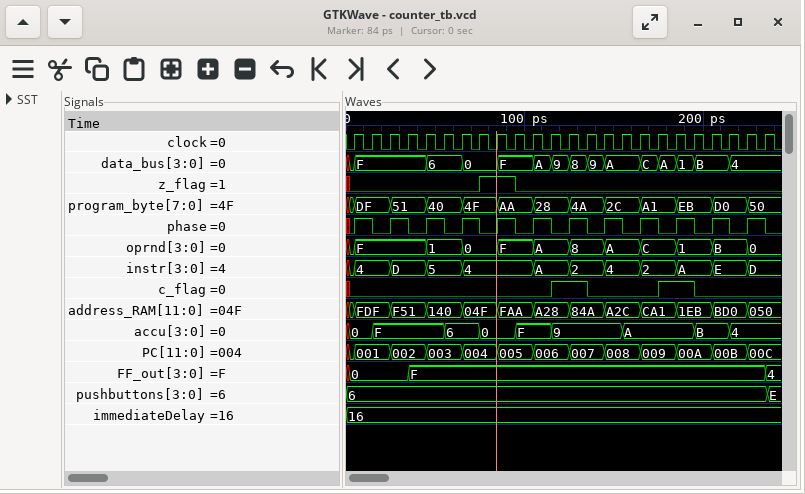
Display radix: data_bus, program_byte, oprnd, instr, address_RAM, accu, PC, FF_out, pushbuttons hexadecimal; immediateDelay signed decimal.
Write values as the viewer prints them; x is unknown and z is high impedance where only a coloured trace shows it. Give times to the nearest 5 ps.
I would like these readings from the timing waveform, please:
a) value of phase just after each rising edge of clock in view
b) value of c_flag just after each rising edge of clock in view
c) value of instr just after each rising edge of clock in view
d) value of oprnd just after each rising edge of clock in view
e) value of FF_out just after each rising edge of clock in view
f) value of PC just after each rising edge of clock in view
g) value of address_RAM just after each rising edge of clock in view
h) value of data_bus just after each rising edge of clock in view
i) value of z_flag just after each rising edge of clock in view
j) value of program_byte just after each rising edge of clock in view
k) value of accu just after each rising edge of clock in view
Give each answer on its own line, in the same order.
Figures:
1 0 1 0 1 0 1 0 1 0 1 0 1 0 1 0 1 0 1 0 1 0 1 0
0 0 0 0 0 0 0 0 0 0 0 1 1 0 0 0 0 1 1 0 0 0 0 0
4, 4, D, D, 5, 5, 4, 4, 4, 4, A, A, 2, 2, 4, 4, 2, 2, A, A, E, E, D, D
F, F, F, F, 1, 1, 0, 0, F, F, A, A, 8, 8, A, A, C, C, 1, 1, B, B, 0, 0
0, 0, 0, F, F, F, F, F, F, F, F, F, F, F, F, F, F, F, F, F, F, F, F, 4
001, 001, 002, 002, 003, 003, 004, 004, 005, 005, 006, 006, 007, 007, 008, 008, 009, 009, 00A, 00A, 00B, 00B, 00C, 00C
FDF, FDF, F51, F51, 140, 140, 04F, 04F, FAA, FAA, A28, A28, 84A, 84A, A2C, A2C, CA1, CA1, 1EB, 1EB, BD0, BD0, 050, 050
F, F, F, F, 6, 6, 0, 0, F, F, A, 9, 8, 9, A, A, C, A, 1, B, B, 4, 4, 4
0 0 0 0 0 0 0 1 1 0 0 0 0 0 0 0 0 0 0 0 0 0 0 0
DF, DF, 51, 51, 40, 40, 4F, 4F, AA, AA, 28, 28, 4A, 4A, 2C, 2C, A1, A1, EB, EB, D0, D0, 50, 50
0, F, F, F, F, 6, 6, 0, 0, F, F, 9, 9, 9, 9, A, A, A, A, B, B, 4, 4, 4
